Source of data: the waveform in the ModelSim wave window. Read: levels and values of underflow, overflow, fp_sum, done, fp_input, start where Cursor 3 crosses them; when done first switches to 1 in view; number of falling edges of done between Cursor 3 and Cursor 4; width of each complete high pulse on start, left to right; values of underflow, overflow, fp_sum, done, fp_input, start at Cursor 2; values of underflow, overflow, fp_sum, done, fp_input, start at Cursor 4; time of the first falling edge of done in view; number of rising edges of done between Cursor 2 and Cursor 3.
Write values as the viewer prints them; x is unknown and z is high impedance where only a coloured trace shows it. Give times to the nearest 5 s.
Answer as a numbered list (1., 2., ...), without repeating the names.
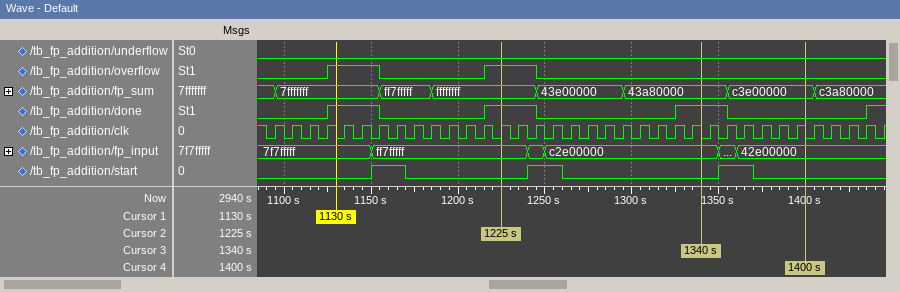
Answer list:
1. underflow=0, overflow=0, fp_sum=43a80000, done=1, fp_input=c2e00000, start=0
2. 1125 s
3. 1
4. 20 s, 20 s, 20 s
5. underflow=0, overflow=1, fp_sum=ffffffff, done=1, fp_input=ff7fffff, start=0
6. underflow=0, overflow=0, fp_sum=c3e00000, done=0, fp_input=42e00000, start=0
7. 1155 s
8. 1
